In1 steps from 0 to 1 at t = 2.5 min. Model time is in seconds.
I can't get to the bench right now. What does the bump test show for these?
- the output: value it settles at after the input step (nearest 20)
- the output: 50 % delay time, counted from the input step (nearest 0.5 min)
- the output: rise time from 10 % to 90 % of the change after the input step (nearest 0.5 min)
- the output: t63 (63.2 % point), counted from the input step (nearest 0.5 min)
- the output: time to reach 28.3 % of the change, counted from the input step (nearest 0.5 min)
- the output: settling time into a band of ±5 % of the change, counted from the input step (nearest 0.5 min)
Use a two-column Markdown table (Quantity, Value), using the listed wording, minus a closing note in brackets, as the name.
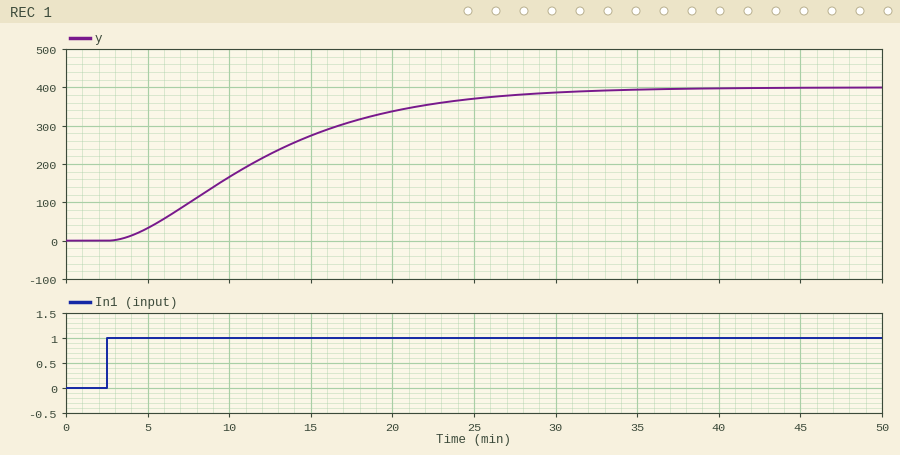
| Quantity | Value |
|---|---|
| the output: value it settles at after the input step | 400 |
| the output: 50 % delay time, counted from the input step | 9.0 min |
| the output: rise time from 10 % to 90 % of the change after the input step | 17.5 min |
| the output: t63 (63.2 % point), counted from the input step | 11.5 min |
| the output: time to reach 28.3 % of the change, counted from the input step | 5.5 min |
| the output: settling time into a band of ±5 % of the change, counted from the input step | 25.0 min |
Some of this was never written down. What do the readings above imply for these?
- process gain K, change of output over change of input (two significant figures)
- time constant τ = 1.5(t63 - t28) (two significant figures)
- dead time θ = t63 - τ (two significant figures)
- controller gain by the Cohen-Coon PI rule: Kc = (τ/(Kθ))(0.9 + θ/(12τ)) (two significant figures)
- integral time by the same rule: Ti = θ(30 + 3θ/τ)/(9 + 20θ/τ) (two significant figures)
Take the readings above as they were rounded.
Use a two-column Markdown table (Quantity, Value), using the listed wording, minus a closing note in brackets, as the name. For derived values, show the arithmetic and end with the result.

| Quantity | Value |
|---|---|
| process gain K, change of output over change of input | (400 - 0) / 1 = 400 |
| time constant τ = 1.5(t63 - t28) | 1.5 × (11.5 - 5.5) = 9.0 min |
| dead time θ = t63 - τ | 11.5 - 9 = 2.5 min |
| controller gain by the Cohen-Coon PI rule: Kc = (τ/(Kθ))(0.9 + θ/(12τ)) | 9 / (400 × 2.5) × (0.9 + 2.5 / (12 × 9)) = 0.0083 |
| integral time by the same rule: Ti = θ(30 + 3θ/τ)/(9 + 20θ/τ) | 2.5 × (30 + 3 × 2.5 / 9) / (9 + 20 × 2.5 / 9) = 5.3 min |
